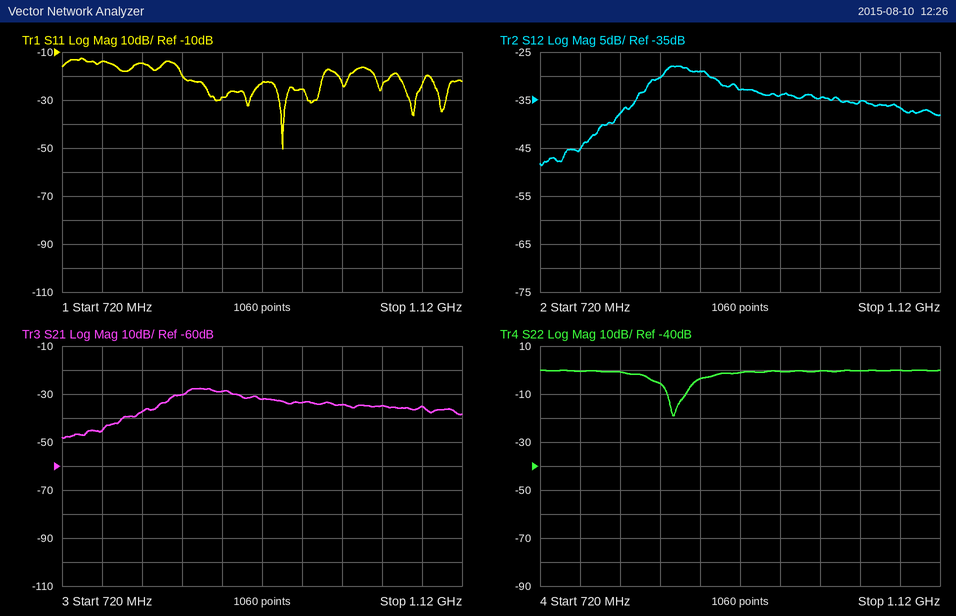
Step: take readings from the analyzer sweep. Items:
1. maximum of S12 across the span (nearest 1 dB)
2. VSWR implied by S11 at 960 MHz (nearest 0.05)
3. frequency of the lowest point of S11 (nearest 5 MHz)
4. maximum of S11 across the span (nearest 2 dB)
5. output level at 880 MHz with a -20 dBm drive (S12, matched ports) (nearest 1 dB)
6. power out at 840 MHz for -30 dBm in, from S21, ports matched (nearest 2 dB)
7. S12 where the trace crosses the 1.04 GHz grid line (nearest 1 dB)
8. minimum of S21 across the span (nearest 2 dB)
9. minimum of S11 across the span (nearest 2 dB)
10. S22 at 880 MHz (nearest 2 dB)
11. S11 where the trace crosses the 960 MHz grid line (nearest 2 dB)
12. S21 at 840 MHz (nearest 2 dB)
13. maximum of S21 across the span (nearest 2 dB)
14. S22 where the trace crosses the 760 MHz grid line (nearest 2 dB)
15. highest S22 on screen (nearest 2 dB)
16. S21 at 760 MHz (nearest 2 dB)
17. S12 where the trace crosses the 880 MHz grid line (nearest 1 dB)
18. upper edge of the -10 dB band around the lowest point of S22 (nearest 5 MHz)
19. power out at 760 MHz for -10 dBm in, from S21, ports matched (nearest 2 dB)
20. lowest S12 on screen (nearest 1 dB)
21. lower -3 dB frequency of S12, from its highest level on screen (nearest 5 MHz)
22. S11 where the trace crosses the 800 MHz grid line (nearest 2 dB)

-28 dB
1.10
940 MHz
-12 dB
-49 dBm
-60 dBm
-35 dB
-48 dB
-50 dB
-4 dB
-26 dB
-30 dB
-28 dB
0 dB
0 dB
-46 dB
-29 dB
865 MHz
-56 dBm
-49 dB
830 MHz
-14 dB
